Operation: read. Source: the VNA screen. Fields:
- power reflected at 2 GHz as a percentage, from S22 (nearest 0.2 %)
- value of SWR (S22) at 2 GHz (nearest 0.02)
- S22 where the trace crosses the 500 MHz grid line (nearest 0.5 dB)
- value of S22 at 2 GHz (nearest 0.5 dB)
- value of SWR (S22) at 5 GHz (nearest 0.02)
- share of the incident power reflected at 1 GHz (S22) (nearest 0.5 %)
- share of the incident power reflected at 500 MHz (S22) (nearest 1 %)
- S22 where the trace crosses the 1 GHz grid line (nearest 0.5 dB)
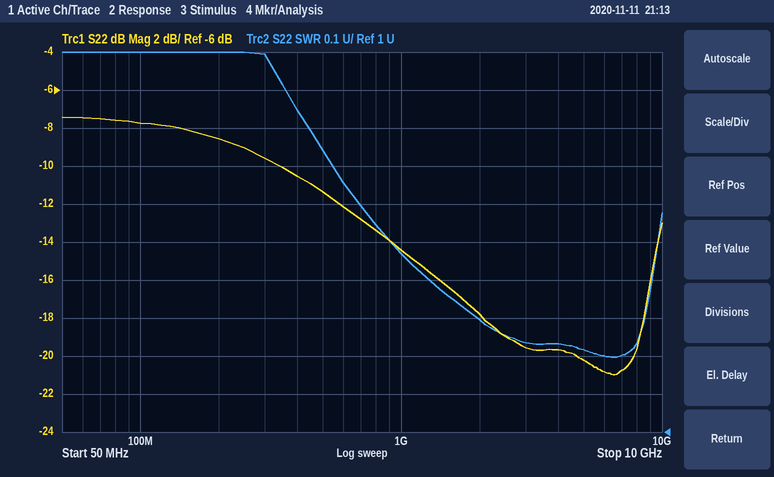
1.6 %
1.30
-11.5 dB
-18.0 dB
1.22
3.5 %
7 %
-14.5 dB
